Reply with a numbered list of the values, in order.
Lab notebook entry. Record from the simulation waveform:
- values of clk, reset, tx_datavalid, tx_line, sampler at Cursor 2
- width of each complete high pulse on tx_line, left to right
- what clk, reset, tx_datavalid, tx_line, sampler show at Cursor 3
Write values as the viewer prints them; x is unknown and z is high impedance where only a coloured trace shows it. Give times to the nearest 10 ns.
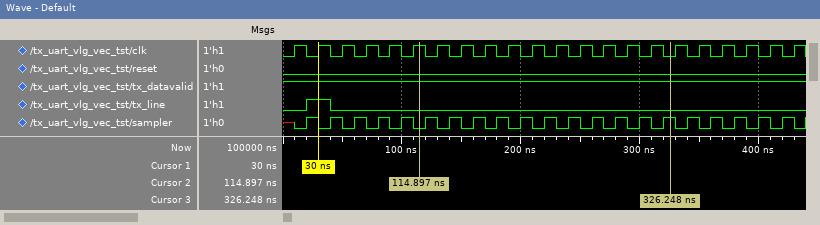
1. clk=1, reset=0, tx_datavalid=1, tx_line=0, sampler=0
2. 20 ns
3. clk=0, reset=0, tx_datavalid=1, tx_line=0, sampler=1
